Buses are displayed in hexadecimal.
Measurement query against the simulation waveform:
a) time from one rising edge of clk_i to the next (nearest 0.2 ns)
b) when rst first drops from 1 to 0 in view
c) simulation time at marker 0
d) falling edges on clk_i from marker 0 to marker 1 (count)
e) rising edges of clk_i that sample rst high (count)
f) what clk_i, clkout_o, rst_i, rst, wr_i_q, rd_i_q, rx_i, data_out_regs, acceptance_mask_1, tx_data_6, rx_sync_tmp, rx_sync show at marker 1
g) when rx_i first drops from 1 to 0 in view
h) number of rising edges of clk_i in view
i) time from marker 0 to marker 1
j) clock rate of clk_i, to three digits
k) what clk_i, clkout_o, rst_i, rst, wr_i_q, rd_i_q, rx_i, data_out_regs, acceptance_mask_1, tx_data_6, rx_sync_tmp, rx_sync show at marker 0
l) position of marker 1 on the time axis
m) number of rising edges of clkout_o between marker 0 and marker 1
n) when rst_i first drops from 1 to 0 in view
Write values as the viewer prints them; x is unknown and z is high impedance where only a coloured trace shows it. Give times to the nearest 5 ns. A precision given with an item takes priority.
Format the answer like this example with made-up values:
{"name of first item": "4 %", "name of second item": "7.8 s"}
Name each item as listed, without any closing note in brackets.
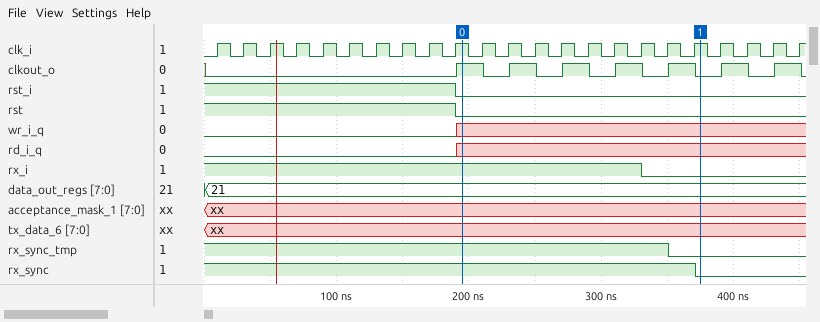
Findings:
{"time from one rising edge of clk_i to the next": "20 ns", "when rst first drops from 1 to 0 in view": "190 ns", "simulation time at marker 0": "195 ns", "falling edges on clk_i from marker 0 to marker 1": "9", "rising edges of clk_i that sample rst high": "10", "what clk_i, clkout_o, rst_i, rst, wr_i_q, rd_i_q, rx_i, data_out_regs, acceptance_mask_1, tx_data_6, rx_sync_tmp, rx_sync show at marker 1": "clk_i=1, clkout_o=0, rst_i=0, rst=0, wr_i_q=x, rd_i_q=x, rx_i=0, data_out_regs=21, acceptance_mask_1=xx, tx_data_6=xx, rx_sync_tmp=0, rx_sync=0", "when rx_i first drops from 1 to 0 in view": "330 ns", "number of rising edges of clk_i in view": "23", "time from marker 0 to marker 1": "180 ns", "clock rate of clk_i, to three digits": "50.0 MHz", "what clk_i, clkout_o, rst_i, rst, wr_i_q, rd_i_q, rx_i, data_out_regs, acceptance_mask_1, tx_data_6, rx_sync_tmp, rx_sync show at marker 0": "clk_i=1, clkout_o=1, rst_i=0, rst=0, wr_i_q=x, rd_i_q=x, rx_i=1, data_out_regs=21, acceptance_mask_1=xx, tx_data_6=xx, rx_sync_tmp=1, rx_sync=1", "position of marker 1 on the time axis": "375 ns", "number of rising edges of clkout_o between marker 0 and marker 1": "4", "when rst_i first drops from 1 to 0 in view": "190 ns"}
